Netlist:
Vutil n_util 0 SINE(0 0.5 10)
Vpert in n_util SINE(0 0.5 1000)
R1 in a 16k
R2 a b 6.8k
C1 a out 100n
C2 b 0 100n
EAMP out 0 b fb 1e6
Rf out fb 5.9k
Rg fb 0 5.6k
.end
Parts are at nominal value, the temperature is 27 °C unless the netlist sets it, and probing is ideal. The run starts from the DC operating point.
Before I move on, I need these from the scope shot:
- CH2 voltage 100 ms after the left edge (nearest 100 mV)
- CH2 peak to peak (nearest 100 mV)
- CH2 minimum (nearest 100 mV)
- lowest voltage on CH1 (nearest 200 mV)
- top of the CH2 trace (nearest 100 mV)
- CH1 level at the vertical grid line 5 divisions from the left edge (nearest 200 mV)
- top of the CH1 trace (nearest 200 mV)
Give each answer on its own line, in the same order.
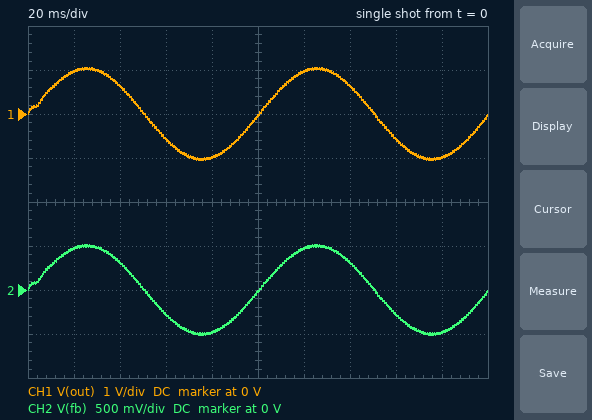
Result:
0 V
1.0 V
-500 mV
-1.0 V
500 mV
0 V
1.0 V
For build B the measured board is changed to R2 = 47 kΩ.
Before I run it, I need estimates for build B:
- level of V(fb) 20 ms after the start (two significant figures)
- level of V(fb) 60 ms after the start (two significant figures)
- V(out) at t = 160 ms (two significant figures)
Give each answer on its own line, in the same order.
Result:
410 mV
-160 mV
-340 mV
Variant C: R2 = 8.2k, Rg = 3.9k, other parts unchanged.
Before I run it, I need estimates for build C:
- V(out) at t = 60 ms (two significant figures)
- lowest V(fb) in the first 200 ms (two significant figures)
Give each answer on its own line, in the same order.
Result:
-670 mV
-540 mV
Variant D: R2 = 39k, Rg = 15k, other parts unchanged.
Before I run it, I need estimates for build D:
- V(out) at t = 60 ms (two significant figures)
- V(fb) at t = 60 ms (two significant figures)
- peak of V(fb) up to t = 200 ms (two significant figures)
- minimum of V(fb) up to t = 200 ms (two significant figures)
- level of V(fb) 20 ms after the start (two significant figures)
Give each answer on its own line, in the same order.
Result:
-220 mV
-160 mV
490 mV
-490 mV
400 mV
